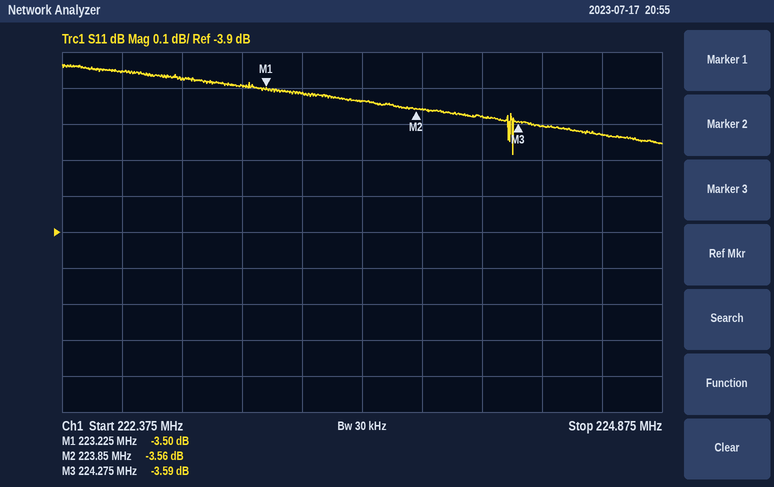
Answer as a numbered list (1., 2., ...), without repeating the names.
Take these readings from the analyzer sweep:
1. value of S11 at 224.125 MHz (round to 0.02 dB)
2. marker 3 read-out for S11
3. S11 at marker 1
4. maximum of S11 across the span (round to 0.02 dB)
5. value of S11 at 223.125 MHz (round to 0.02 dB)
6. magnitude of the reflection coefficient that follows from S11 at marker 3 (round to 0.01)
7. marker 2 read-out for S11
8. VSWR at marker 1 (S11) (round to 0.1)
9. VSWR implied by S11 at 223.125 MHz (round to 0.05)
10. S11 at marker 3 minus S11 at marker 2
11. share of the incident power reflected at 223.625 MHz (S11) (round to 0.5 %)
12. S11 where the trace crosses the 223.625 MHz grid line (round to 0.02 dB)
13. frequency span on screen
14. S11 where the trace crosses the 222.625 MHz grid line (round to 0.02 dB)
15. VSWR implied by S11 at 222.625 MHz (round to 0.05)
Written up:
1. -3.58 dB
2. -3.59 dB
3. -3.50 dB
4. -3.44 dB
5. -3.50 dB
6. 0.66
7. -3.56 dB
8. 5.0
9. 5.05
10. -0.03 dB
11. 44.5 %
12. -3.54 dB
13. 2.5 MHz
14. -3.46 dB
15. 5.10
